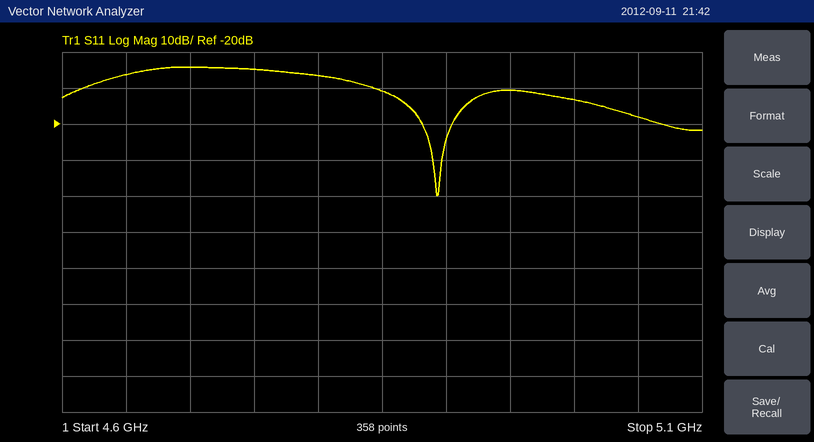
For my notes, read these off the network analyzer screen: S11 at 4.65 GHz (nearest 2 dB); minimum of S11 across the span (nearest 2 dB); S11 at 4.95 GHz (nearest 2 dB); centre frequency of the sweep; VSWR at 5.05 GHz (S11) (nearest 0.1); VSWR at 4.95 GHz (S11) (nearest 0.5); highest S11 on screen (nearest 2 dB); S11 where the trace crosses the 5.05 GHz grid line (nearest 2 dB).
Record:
-6 dB
-40 dB
-10 dB
4.85 GHz
1.3
2.0
-4 dB
-18 dB
